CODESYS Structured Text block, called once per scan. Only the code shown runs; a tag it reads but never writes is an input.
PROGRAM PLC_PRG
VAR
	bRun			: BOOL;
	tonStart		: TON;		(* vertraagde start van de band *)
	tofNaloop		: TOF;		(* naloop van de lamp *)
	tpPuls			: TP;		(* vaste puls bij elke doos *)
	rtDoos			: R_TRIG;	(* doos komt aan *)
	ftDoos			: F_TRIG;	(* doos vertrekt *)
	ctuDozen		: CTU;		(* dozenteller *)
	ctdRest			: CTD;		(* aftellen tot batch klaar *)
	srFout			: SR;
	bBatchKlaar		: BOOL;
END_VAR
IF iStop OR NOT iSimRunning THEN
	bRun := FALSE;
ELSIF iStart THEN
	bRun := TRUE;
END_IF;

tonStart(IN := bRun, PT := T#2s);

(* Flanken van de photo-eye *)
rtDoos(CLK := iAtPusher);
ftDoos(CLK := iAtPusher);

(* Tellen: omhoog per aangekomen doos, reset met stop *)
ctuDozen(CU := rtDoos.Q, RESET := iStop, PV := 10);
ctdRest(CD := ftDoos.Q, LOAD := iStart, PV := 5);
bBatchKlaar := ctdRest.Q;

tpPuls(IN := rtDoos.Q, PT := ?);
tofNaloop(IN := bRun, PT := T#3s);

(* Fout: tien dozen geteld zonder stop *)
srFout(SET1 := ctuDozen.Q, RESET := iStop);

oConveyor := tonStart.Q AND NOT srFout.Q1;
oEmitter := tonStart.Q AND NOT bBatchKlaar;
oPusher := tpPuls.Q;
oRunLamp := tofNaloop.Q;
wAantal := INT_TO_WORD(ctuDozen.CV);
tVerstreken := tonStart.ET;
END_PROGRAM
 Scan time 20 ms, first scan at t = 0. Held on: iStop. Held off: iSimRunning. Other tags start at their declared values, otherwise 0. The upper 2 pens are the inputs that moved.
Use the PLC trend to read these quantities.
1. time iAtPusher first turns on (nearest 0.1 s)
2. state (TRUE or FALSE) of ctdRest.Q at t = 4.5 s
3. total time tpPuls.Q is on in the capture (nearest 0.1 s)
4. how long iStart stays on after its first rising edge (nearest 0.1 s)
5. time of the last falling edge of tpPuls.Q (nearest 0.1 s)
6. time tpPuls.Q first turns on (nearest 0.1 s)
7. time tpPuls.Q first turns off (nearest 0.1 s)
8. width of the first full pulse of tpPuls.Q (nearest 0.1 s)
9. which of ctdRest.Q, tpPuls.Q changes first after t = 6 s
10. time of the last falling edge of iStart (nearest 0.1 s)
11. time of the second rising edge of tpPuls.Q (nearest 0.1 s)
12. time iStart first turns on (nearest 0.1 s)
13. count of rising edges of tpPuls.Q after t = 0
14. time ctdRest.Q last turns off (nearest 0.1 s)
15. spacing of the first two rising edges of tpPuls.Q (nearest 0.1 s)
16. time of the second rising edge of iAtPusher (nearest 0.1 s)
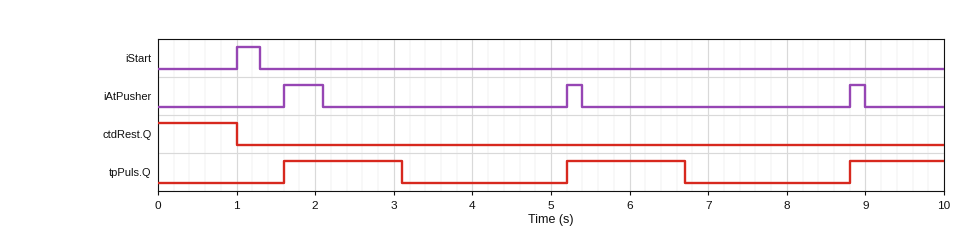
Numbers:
1.6 s
FALSE
4.2 s
0.3 s
6.7 s
1.6 s
3.1 s
1.5 s
tpPuls.Q
1.3 s
5.2 s
1.0 s
3
1.0 s
3.6 s
5.2 s
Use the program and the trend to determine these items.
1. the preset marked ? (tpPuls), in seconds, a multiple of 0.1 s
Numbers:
1.5 s
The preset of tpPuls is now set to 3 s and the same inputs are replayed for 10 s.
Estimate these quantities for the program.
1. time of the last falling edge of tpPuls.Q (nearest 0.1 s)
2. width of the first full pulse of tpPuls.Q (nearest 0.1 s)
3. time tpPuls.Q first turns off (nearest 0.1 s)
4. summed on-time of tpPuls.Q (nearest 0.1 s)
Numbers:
8.2 s
3.0 s
4.6 s
7.2 s
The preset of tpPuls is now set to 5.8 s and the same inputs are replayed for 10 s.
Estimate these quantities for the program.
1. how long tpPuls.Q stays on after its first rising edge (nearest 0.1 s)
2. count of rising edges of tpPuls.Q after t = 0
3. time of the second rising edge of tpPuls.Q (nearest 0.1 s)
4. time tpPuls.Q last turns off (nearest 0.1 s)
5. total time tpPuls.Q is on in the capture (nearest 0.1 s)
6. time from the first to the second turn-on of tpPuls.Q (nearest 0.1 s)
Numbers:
5.8 s
2
8.8 s
7.4 s
7.0 s
7.2 s
